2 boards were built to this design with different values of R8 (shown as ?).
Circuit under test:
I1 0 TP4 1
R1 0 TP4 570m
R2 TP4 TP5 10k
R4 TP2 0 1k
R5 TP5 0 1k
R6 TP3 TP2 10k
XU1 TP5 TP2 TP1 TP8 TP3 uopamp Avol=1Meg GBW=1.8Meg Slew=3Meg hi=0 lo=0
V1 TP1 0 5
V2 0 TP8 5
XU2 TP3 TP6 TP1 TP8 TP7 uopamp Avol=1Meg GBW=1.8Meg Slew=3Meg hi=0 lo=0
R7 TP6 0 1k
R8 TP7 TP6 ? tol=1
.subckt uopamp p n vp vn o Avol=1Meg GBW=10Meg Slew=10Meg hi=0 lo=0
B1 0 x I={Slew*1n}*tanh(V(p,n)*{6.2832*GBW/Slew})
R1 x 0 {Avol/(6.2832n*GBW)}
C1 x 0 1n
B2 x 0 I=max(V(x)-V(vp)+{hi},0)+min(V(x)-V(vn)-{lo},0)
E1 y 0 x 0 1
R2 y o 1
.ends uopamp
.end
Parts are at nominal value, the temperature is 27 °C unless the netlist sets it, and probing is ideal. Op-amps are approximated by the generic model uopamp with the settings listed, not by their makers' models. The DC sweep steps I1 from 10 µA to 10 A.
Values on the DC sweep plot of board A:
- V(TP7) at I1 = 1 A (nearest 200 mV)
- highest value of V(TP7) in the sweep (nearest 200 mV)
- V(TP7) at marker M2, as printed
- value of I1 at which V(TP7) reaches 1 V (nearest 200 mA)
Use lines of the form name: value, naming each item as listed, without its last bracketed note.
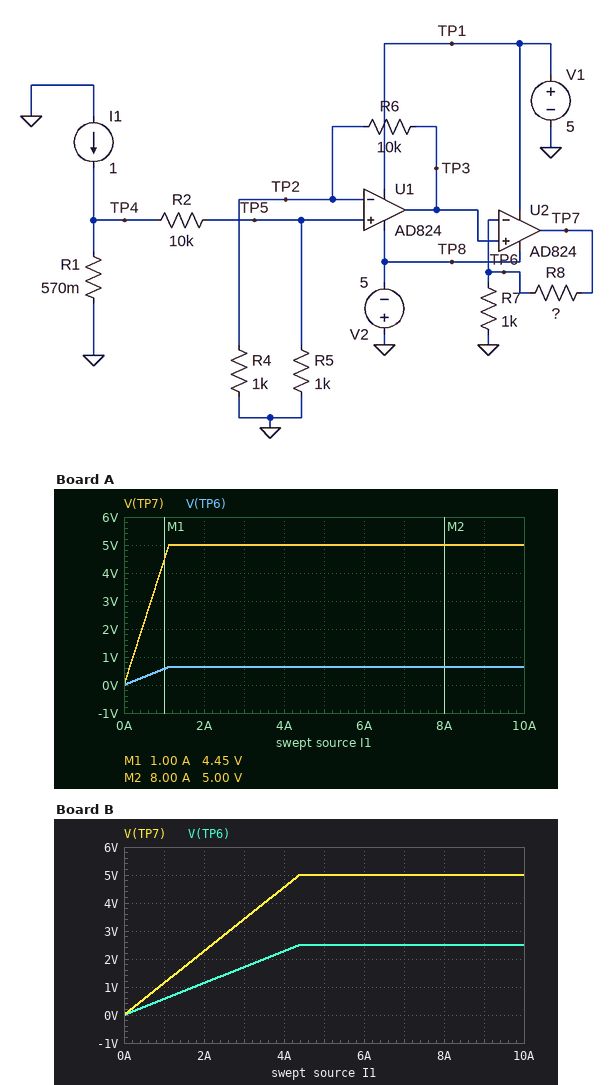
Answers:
V(TP7) at I1 = 1 A: 4.4 V
highest value of V(TP7) in the sweep: 5.0 V
V(TP7) at marker M2, as printed: 5.00 V
value of I1 at which V(TP7) reaches 1 V: 200 mA
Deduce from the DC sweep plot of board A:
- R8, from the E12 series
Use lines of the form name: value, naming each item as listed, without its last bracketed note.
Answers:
R8, from the E12 series: 6.8 kΩ
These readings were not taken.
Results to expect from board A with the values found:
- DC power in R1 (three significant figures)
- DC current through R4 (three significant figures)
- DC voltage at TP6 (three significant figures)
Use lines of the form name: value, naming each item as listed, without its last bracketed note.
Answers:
DC power in R1: 570 mW
DC current through R4: 51.8 µA
DC voltage at TP6: 570 mV
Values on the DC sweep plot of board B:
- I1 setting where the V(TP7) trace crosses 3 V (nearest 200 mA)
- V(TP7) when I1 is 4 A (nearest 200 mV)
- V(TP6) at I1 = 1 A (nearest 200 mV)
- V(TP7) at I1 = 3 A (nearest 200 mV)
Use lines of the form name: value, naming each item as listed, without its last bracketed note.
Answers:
I1 setting where the V(TP7) trace crosses 3 V: 2.6 A
V(TP7) when I1 is 4 A: 4.6 V
V(TP6) at I1 = 1 A: 600 mV
V(TP7) at I1 = 3 A: 3.4 V
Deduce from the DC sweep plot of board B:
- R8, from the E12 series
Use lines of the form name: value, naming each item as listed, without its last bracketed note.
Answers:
R8, from the E12 series: 1 kΩ
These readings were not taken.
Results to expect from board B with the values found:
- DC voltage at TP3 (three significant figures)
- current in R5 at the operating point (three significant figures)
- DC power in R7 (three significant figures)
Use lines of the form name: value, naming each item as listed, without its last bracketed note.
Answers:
DC voltage at TP3: 570 mV
current in R5 at the operating point: 51.8 µA
DC power in R7: 325 µW
